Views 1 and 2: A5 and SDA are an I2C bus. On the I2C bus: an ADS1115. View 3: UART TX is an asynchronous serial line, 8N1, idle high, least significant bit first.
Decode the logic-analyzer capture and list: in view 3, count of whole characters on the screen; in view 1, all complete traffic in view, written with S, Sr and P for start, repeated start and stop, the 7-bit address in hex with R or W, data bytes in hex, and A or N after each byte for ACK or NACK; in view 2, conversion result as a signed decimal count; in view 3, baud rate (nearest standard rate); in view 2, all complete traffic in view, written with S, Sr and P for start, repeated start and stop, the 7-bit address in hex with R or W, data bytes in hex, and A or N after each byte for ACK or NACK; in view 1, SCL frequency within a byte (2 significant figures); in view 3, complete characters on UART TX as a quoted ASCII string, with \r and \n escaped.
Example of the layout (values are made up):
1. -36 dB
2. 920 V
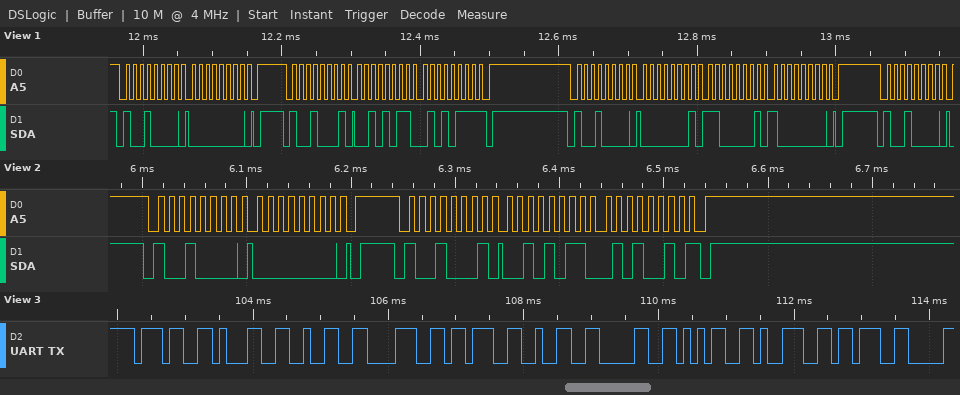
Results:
1. 10
2. S 48W A 00 A P S 48R A 2B A 57 N P S 48W A 01 A C1 A 80 A P S 48W A
3. 11090
4. 9600 baud
5. S 48W A 00 A P S 48R A 2B A 52 N P
6. 100 kHz
7. "7128;2059;"
